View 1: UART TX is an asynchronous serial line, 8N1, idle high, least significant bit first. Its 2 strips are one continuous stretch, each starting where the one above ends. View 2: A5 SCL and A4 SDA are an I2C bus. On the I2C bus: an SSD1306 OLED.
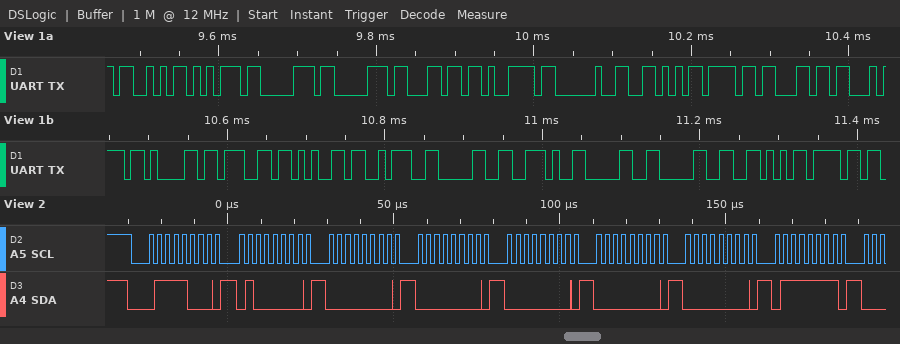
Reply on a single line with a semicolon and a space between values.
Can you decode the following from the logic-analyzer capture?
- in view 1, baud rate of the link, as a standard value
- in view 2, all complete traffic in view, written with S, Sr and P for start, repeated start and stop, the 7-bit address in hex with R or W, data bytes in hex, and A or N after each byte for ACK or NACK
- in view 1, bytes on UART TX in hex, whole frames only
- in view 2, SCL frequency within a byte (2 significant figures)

115200 baud; S 3CW A 40 A 00 A 00 A 00 A 00 A 00 A 7F A; 53 75 70 70 6C 79 20 56 6F 6C 74 61 67 65 3A 30 2E 30 30 56 6F; 400 kHz
